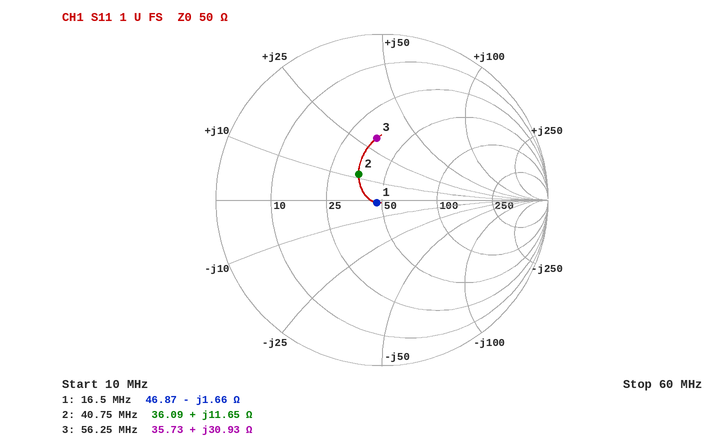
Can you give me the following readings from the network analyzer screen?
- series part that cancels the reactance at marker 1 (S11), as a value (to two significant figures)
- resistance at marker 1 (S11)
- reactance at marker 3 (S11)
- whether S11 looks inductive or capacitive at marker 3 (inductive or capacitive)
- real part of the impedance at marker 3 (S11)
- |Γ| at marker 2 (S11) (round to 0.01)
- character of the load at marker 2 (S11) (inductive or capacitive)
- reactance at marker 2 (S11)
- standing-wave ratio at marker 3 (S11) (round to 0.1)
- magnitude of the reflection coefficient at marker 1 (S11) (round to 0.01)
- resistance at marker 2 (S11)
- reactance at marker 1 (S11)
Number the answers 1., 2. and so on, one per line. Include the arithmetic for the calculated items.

1. L = 1.66 Ω/(2π × 16.5 MHz) ≈ 16 nH
2. 46.87 Ω
3. +30.93 Ω
4. inductive
5. 35.73 Ω
6. 0.21
7. inductive
8. +11.65 Ω
9. 2.2
10. 0.04
11. 36.09 Ω
12. -1.66 Ω
